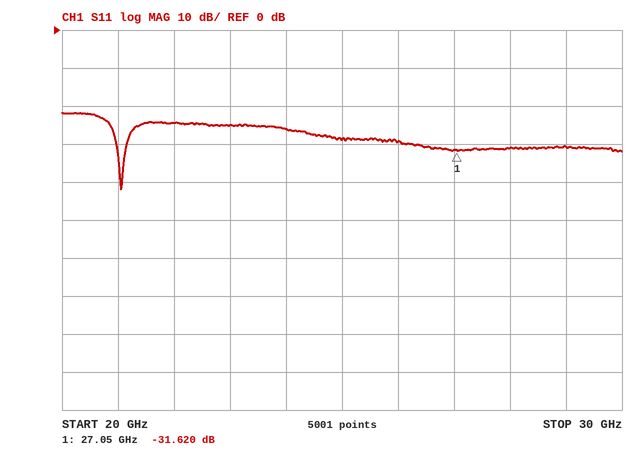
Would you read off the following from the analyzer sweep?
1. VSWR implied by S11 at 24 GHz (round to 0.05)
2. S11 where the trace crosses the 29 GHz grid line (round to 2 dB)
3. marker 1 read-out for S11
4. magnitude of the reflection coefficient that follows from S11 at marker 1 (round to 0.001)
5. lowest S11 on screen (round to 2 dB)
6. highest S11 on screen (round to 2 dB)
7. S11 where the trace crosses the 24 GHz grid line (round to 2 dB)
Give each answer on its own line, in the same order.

1.10
-30 dB
-31.620 dB
0.026
-42 dB
-22 dB
-26 dB
